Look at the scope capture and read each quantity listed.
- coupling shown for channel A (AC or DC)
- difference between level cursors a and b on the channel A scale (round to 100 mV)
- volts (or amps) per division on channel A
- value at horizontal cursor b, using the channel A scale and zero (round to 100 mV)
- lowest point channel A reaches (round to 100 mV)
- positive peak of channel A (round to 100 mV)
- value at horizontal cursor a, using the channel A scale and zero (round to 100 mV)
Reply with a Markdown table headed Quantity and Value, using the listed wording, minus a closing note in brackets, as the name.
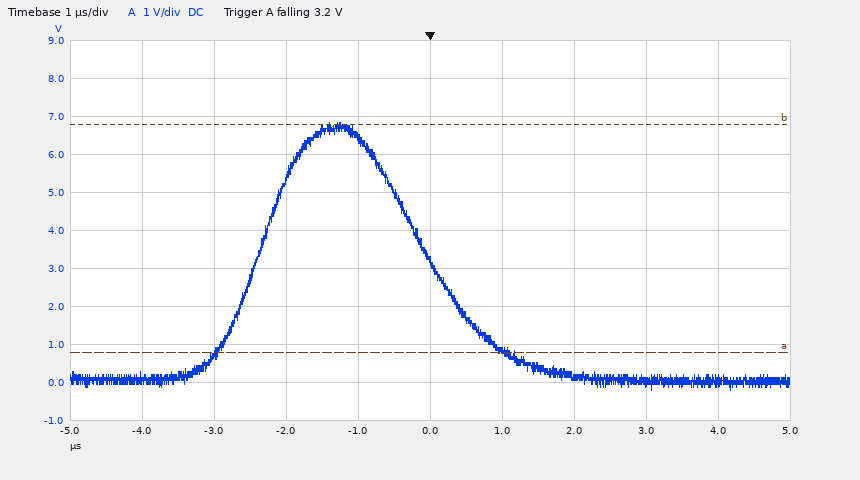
| Quantity | Value |
|---|---|
| coupling shown for channel A | DC |
| difference between level cursors a and b on the channel A scale | 6.0 V |
| volts (or amps) per division on channel A | 1 V |
| value at horizontal cursor b, using the channel A scale and zero | 6.8 V |
| lowest point channel A reaches | -200 mV |
| positive peak of channel A | 6.8 V |
| value at horizontal cursor a, using the channel A scale and zero | 800 mV |
